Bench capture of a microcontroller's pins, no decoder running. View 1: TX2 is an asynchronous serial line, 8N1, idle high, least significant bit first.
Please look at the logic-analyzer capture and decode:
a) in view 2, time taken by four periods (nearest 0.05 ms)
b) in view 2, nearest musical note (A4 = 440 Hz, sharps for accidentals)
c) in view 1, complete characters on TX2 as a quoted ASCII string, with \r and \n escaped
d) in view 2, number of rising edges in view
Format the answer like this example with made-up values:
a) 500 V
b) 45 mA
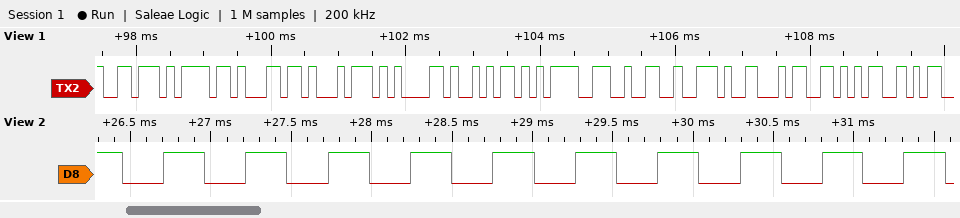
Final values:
a) 2.05 ms
b) B6
c) "voltaj=2.45"
d) 10
